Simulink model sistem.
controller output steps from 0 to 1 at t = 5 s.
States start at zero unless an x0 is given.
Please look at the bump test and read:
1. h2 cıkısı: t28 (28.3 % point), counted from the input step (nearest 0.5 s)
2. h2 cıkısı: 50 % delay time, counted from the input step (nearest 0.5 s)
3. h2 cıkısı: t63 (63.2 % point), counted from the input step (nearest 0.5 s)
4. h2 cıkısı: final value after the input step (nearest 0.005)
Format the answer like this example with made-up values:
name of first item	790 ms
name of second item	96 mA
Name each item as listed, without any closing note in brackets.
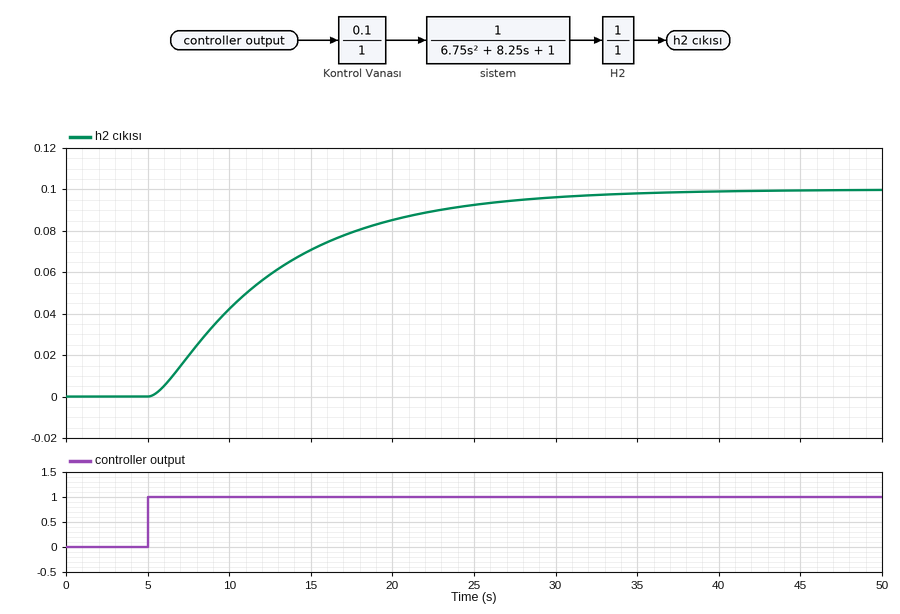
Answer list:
h2 cıkısı: t28 (28.3 % point), counted from the input step	3.5 s
h2 cıkısı: 50 % delay time, counted from the input step	6.0 s
h2 cıkısı: t63 (63.2 % point), counted from the input step	8.5 s
h2 cıkısı: final value after the input step	0.100
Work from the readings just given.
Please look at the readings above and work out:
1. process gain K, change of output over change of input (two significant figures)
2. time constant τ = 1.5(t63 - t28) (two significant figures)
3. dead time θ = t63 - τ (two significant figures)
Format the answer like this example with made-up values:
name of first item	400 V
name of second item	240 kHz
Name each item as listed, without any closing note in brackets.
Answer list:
process gain K, change of output over change of input	0.10
time constant τ = 1.5(t63 - t28)	7.5 s
dead time θ = t63 - τ	1.0 s
